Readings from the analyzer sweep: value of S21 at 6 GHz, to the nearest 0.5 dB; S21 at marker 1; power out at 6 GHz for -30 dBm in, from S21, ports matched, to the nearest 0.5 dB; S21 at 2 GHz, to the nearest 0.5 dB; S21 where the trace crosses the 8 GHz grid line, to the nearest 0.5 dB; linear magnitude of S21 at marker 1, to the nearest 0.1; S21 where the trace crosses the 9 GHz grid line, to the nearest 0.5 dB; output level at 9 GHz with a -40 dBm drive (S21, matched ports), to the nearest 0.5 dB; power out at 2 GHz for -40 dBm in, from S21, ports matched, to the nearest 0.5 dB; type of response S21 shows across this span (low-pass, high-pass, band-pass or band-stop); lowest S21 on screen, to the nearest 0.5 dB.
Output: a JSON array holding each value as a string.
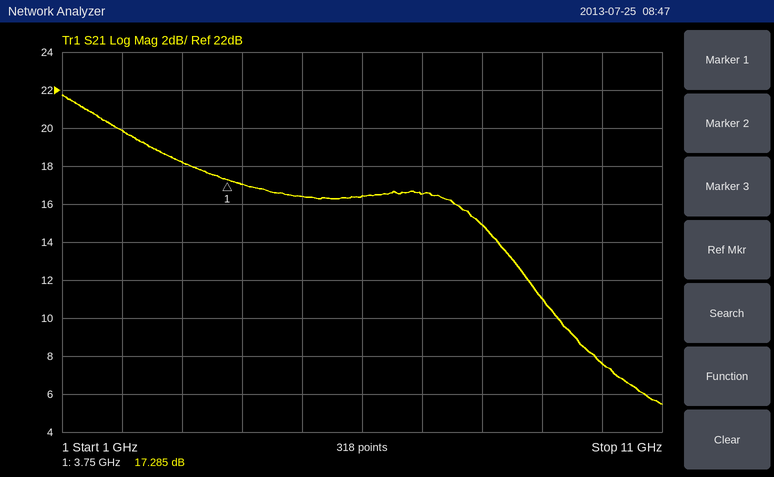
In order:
["16.5 dB", "17.285 dB", "-13.5 dBm", "20.0 dB", "15.0 dB", "7.3", "11.0 dB", "-29.0 dBm", "-20.0 dBm", "low-pass", "5.5 dB"]
